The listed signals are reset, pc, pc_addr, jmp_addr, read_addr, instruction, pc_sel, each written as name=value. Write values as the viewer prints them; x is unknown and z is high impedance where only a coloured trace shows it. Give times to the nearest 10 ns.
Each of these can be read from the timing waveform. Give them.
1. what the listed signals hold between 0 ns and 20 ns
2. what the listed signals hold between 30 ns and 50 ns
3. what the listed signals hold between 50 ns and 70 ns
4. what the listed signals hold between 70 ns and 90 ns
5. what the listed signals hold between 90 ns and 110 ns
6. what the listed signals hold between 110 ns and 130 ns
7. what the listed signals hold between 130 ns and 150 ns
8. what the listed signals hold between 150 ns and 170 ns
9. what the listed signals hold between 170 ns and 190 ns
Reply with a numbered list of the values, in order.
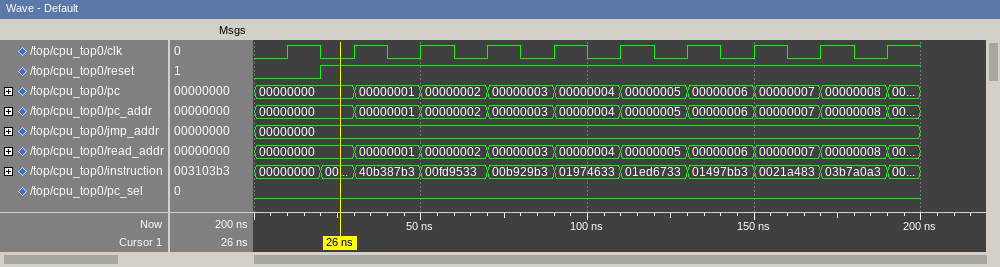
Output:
1. reset=0, pc=00000000, pc_addr=00000000, jmp_addr=00000000, read_addr=00000000, instruction=00000000, pc_sel=0
2. reset=1, pc=00000001, pc_addr=00000001, jmp_addr=00000000, read_addr=00000001, instruction=40b387b3, pc_sel=0
3. reset=1, pc=00000002, pc_addr=00000002, jmp_addr=00000000, read_addr=00000002, instruction=00fd9533, pc_sel=0
4. reset=1, pc=00000003, pc_addr=00000003, jmp_addr=00000000, read_addr=00000003, instruction=00b929b3, pc_sel=0
5. reset=1, pc=00000004, pc_addr=00000004, jmp_addr=00000000, read_addr=00000004, instruction=01974633, pc_sel=0
6. reset=1, pc=00000005, pc_addr=00000005, jmp_addr=00000000, read_addr=00000005, instruction=01ed6733, pc_sel=0
7. reset=1, pc=00000006, pc_addr=00000006, jmp_addr=00000000, read_addr=00000006, instruction=01497bb3, pc_sel=0
8. reset=1, pc=00000007, pc_addr=00000007, jmp_addr=00000000, read_addr=00000007, instruction=0021a483, pc_sel=0
9. reset=1, pc=00000008, pc_addr=00000008, jmp_addr=00000000, read_addr=00000008, instruction=03b7a0a3, pc_sel=0
